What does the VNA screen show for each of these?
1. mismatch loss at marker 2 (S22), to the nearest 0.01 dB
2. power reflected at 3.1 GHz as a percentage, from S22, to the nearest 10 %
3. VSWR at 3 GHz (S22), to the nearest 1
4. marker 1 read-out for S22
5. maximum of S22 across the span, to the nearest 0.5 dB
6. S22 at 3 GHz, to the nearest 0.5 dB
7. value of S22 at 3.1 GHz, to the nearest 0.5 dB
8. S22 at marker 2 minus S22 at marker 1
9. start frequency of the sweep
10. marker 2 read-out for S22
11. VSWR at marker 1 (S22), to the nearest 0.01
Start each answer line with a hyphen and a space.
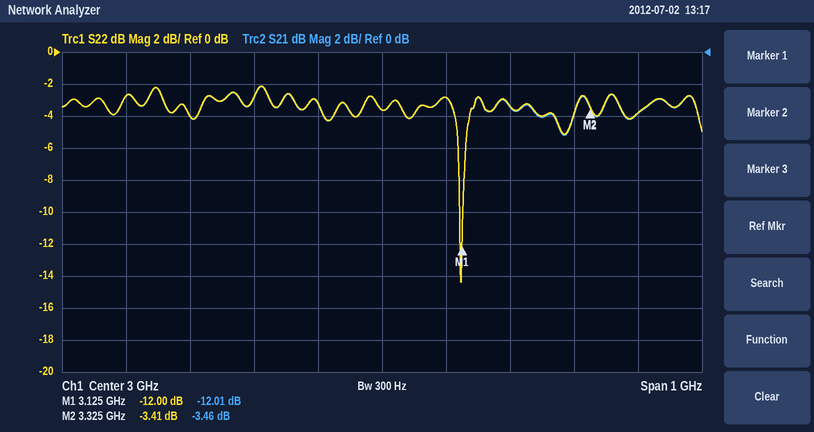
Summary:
- 2.64 dB
- 50 %
- 5
- -12.00 dB
- -2.0 dB
- -3.5 dB
- -3.0 dB
- 8.59 dB
- 2.5 GHz
- -3.41 dB
- 1.67
